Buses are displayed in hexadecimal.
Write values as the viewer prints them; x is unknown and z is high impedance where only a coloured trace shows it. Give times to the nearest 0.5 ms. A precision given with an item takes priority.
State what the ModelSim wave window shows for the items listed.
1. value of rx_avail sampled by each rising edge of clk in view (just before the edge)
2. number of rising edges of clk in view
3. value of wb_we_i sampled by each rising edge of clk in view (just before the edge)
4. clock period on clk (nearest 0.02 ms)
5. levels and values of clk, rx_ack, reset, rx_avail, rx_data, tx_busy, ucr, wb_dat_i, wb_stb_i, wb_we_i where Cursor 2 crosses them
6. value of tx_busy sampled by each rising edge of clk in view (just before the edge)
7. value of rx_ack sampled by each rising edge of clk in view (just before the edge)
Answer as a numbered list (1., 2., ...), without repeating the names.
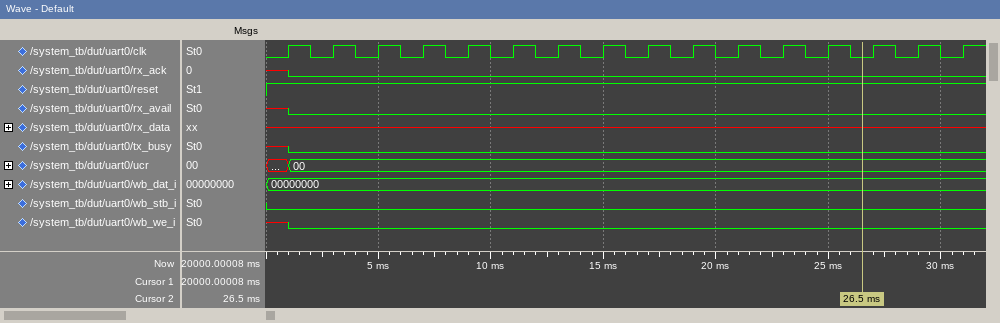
1. x 0 0 0 0 0 0 0 0 0 0 0 0 0 0 0
2. 16
3. x 0 0 0 0 0 0 0 0 0 0 0 0 0 0 0
4. 2 ms
5. clk=0, rx_ack=0, reset=1, rx_avail=0, rx_data=x, tx_busy=0, ucr=00, wb_dat_i=00000000, wb_stb_i=0, wb_we_i=0
6. x 0 0 0 0 0 0 0 0 0 0 0 0 0 0 0
7. x 0 0 0 0 0 0 0 0 0 0 0 0 0 0 0
